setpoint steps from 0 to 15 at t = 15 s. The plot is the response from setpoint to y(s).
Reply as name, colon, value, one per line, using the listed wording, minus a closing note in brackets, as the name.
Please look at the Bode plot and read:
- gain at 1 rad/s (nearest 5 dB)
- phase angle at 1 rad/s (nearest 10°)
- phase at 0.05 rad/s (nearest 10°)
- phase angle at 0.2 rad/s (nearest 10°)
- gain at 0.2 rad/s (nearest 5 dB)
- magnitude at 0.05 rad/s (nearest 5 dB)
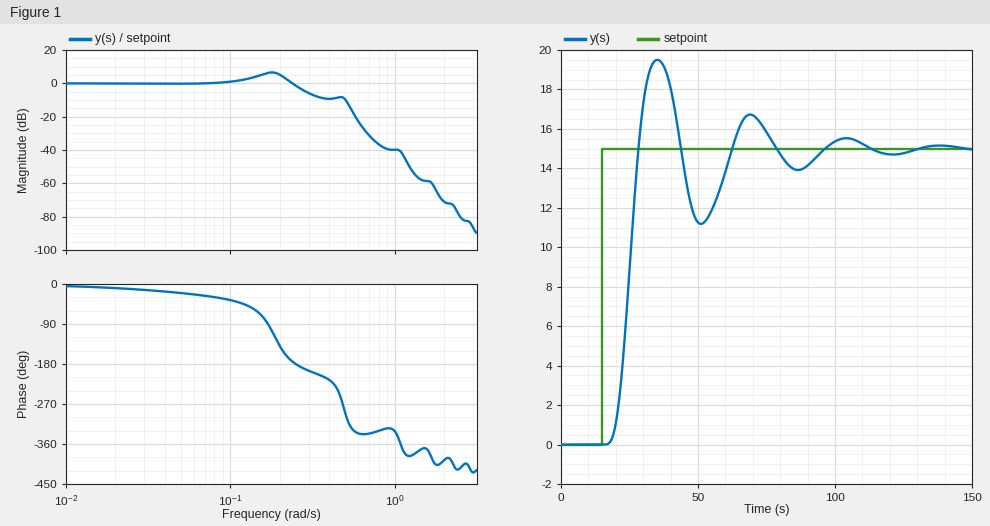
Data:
gain at 1 rad/s: -40 dB
phase angle at 1 rad/s: -330°
phase at 0.05 rad/s: -20°
phase angle at 0.2 rad/s: -140°
gain at 0.2 rad/s: 5 dB
magnitude at 0.05 rad/s: 0 dB
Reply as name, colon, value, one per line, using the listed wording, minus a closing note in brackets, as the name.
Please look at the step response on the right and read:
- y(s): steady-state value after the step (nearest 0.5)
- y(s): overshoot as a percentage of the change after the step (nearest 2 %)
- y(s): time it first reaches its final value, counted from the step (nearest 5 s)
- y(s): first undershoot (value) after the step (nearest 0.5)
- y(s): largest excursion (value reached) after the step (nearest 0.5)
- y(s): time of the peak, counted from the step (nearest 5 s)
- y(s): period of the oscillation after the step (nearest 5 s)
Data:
y(s): steady-state value after the step: 15.0
y(s): overshoot as a percentage of the change after the step: 30 %
y(s): time it first reaches its final value, counted from the step: 15 s
y(s): first undershoot (value) after the step: 11.0
y(s): largest excursion (value reached) after the step: 19.5
y(s): time of the peak, counted from the step: 20 s
y(s): period of the oscillation after the step: 35 s
